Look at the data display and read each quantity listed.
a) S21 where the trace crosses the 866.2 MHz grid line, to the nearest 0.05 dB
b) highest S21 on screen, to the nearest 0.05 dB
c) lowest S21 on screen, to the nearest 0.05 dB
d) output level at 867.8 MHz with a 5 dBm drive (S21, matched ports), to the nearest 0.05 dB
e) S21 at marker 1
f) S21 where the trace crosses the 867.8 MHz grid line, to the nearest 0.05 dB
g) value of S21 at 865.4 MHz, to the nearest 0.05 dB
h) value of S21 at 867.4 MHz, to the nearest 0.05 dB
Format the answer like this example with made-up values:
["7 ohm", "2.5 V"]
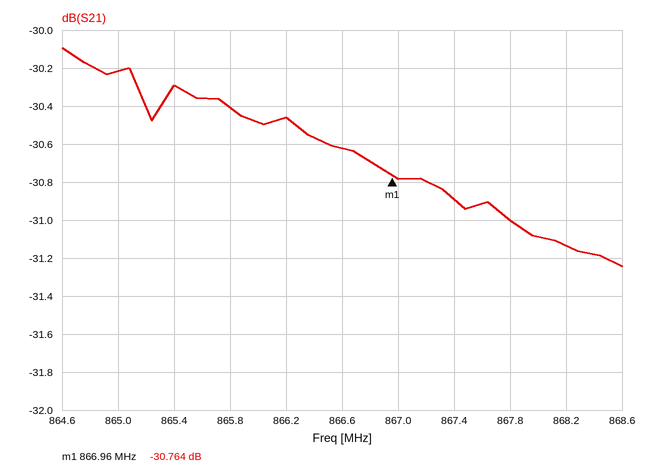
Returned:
["-30.45 dB", "-30.10 dB", "-31.25 dB", "-26.00 dBm", "-30.764 dB", "-31.00 dB", "-30.30 dB", "-30.90 dB"]
